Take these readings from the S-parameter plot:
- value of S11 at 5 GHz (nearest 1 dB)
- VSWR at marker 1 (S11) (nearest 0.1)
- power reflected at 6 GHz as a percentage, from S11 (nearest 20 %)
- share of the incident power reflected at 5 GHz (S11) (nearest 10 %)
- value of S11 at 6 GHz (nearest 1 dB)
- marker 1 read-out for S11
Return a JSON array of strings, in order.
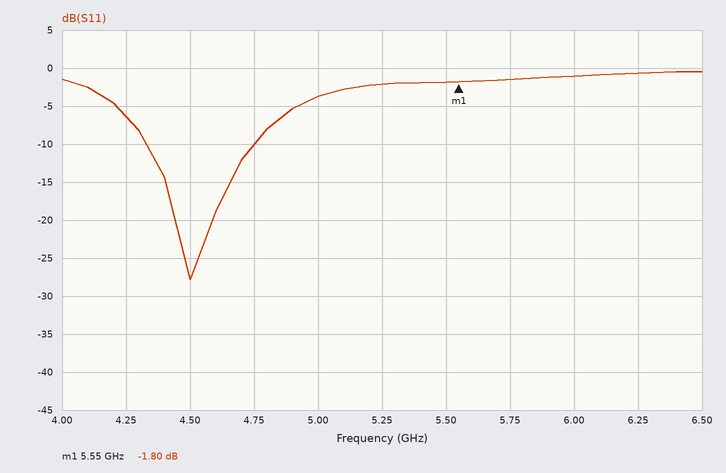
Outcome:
["-4 dB", "9.7", "80 %", "40 %", "-1 dB", "-1.80 dB"]
